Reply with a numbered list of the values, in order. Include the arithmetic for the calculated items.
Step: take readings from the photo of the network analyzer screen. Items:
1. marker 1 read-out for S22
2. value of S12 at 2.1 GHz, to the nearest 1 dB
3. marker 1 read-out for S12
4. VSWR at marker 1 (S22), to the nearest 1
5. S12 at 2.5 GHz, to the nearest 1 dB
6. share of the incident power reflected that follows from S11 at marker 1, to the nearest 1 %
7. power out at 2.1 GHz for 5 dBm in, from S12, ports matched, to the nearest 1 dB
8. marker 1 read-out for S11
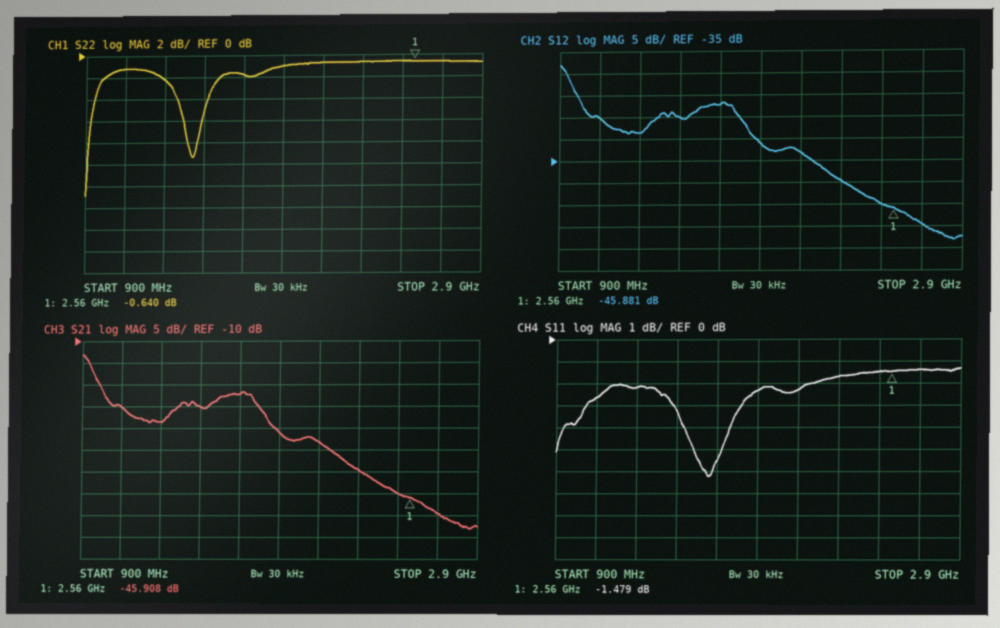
1. -0.640 dB
2. -33 dB
3. -45.881 dB
4. (1 + 0.9290)/(1 − 0.9290) ≈ 27
5. -45 dB
6. 10^(-1.479/10) ≈ 71 %
7. 5 dBm + (-33 dB) = -28 dBm
8. -1.479 dB
